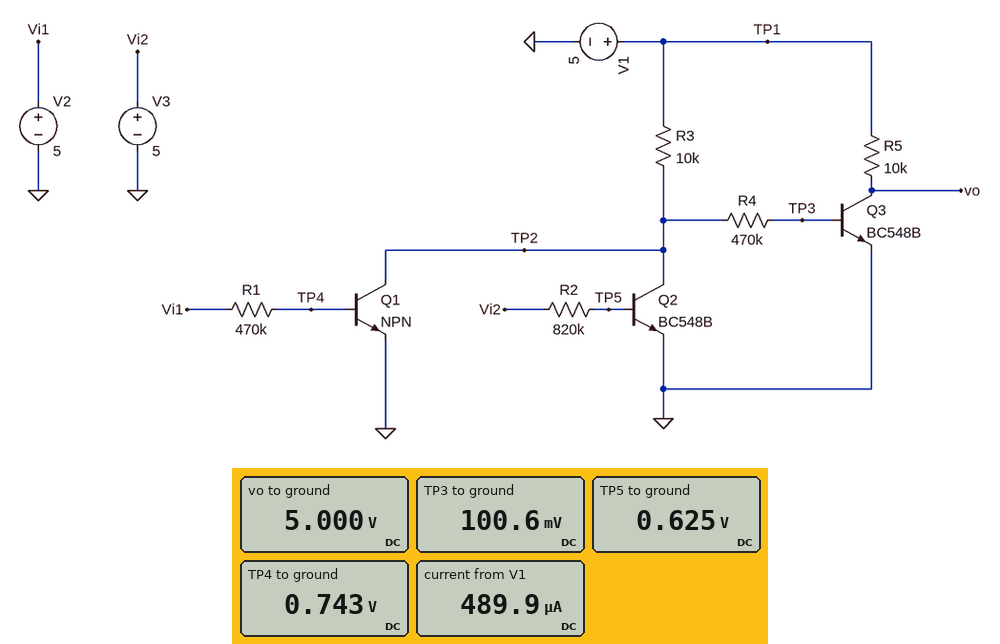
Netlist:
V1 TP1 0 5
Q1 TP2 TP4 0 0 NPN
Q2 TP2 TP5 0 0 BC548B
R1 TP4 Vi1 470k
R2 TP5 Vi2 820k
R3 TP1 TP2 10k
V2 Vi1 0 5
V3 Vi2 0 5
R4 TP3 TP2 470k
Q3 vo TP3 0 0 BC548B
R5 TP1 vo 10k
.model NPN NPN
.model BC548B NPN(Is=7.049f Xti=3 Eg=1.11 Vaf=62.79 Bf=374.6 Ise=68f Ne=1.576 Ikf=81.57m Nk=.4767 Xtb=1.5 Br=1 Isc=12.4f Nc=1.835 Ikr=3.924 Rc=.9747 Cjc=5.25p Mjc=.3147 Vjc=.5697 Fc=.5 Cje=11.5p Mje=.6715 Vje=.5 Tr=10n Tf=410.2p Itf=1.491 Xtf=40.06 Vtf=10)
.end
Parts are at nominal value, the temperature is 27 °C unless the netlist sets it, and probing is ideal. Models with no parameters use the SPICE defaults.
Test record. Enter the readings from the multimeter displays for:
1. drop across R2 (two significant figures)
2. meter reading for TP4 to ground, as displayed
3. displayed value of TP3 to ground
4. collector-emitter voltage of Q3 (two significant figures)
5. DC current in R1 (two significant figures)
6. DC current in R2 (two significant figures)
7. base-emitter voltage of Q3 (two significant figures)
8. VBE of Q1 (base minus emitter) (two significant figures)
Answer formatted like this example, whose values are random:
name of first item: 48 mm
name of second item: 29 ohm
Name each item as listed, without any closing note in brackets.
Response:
drop across R2: 4.4 V
meter reading for TP4 to ground, as displayed: 0.743 V
displayed value of TP3 to ground: 100.6 mV
collector-emitter voltage of Q3: 5.0 V
DC current in R1: 9.1 µA
DC current in R2: 5.3 µA
base-emitter voltage of Q3: 100 mV
VBE of Q1 (base minus emitter): 740 mV
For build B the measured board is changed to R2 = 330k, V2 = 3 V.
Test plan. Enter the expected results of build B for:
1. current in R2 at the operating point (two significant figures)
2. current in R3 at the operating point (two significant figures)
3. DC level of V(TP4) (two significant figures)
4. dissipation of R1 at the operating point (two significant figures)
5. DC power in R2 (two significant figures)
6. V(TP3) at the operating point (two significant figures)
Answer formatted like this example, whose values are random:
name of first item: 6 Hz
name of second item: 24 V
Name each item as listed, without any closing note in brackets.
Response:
current in R2 at the operating point: 13 µA
current in R3 at the operating point: 490 µA
DC level of V(TP4): 720 mV
dissipation of R1 at the operating point: 11 µW
DC power in R2: 58 µW
V(TP3) at the operating point: 92 mV
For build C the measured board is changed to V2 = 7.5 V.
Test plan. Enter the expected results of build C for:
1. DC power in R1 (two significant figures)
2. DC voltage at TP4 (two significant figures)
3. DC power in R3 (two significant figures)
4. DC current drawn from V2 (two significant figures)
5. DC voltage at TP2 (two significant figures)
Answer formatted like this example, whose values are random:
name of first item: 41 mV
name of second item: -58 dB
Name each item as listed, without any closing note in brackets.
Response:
DC power in R1: 97 µW
DC voltage at TP4: 750 mV
DC power in R3: 2.4 mW
DC current drawn from V2: 14 µA
DC voltage at TP2: 91 mV
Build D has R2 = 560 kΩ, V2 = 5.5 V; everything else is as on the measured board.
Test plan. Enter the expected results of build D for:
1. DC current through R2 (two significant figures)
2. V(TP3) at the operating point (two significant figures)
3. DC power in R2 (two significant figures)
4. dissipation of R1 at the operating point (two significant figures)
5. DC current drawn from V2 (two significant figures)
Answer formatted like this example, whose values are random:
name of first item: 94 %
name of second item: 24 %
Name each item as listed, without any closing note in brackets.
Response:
DC current through R2: 7.8 µA
V(TP3) at the operating point: 93 mV
DC power in R2: 34 µW
dissipation of R1 at the operating point: 48 µW
DC current drawn from V2: 10 µA
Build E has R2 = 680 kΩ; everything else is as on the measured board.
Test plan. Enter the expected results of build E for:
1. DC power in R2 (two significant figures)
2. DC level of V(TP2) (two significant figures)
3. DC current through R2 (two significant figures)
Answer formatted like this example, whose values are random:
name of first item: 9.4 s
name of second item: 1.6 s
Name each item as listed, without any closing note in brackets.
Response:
DC power in R2: 28 µW
DC level of V(TP2): 98 mV
DC current through R2: 6.4 µA
